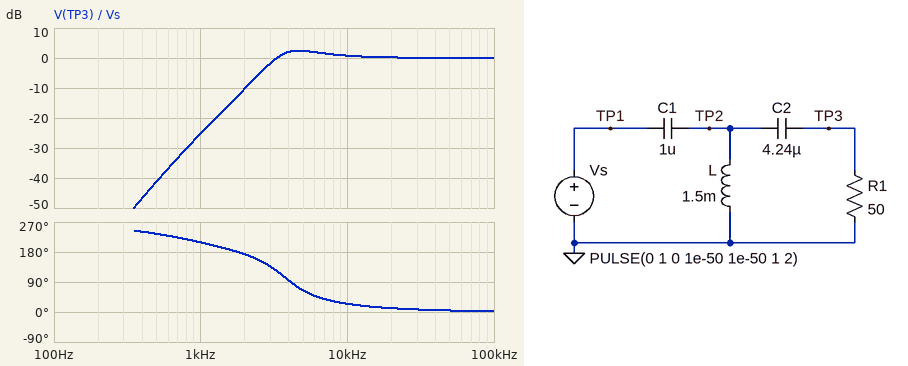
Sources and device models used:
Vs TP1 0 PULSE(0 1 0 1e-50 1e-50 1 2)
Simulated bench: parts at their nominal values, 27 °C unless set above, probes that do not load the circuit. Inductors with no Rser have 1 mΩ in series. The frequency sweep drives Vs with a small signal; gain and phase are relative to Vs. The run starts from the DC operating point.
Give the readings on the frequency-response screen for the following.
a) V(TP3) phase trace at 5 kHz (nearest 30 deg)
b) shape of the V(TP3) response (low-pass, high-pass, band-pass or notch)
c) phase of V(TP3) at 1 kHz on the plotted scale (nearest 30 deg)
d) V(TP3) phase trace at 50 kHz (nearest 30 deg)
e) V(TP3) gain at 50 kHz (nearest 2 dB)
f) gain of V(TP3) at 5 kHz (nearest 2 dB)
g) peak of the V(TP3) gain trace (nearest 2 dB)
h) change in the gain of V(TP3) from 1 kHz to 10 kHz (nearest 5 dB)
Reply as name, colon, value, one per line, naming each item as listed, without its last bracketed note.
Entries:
V(TP3) phase trace at 5 kHz: 60 deg
shape of the V(TP3) response: high-pass
phase of V(TP3) at 1 kHz on the plotted scale: 210 deg
V(TP3) phase trace at 50 kHz: 0 deg
V(TP3) gain at 50 kHz: 0 dB
gain of V(TP3) at 5 kHz: 2 dB
peak of the V(TP3) gain trace: 2 dB
change in the gain of V(TP3) from 1 kHz to 10 kHz: 25 dB
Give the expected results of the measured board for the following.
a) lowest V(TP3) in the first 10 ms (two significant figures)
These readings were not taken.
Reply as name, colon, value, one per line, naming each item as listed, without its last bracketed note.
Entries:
lowest V(TP3) in the first 10 ms: -390 mV
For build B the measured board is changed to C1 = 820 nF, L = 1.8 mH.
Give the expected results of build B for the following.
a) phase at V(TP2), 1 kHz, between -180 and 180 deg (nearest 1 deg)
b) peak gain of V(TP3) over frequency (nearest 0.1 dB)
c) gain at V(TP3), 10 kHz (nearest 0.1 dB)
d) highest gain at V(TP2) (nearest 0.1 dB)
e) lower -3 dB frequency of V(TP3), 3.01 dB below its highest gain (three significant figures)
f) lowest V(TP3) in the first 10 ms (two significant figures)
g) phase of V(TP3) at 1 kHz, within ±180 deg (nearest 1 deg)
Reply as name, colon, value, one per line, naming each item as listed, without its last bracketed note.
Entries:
phase at V(TP2), 1 kHz, between -180 and 180 deg: 170 deg
peak gain of V(TP3) over frequency: 1.1 dB
gain at V(TP3), 10 kHz: 0.5 dB
highest gain at V(TP2): 1.2 dB
lower -3 dB frequency of V(TP3), 3.01 dB below its highest gain: 3.22 kHz
lowest V(TP3) in the first 10 ms: -340 mV
phase of V(TP3) at 1 kHz, within ±180 deg: -153 deg
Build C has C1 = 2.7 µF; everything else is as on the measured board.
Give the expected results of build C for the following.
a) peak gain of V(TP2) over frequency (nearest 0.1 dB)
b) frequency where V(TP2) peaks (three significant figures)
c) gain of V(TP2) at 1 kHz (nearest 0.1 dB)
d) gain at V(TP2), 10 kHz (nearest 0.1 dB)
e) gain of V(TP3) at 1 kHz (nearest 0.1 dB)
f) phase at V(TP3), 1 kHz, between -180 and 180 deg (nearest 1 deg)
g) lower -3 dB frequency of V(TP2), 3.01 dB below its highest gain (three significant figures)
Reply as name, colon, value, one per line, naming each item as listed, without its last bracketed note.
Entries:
peak gain of V(TP2) over frequency: 6.9 dB
frequency where V(TP2) peaks: 2.44 kHz
gain of V(TP2) at 1 kHz: -13.5 dB
gain at V(TP2), 10 kHz: 0.4 dB
gain of V(TP3) at 1 kHz: -15.5 dB
phase at V(TP3), 1 kHz, between -180 and 180 deg: -152 deg
lower -3 dB frequency of V(TP2), 3.01 dB below its highest gain: 2.00 kHz
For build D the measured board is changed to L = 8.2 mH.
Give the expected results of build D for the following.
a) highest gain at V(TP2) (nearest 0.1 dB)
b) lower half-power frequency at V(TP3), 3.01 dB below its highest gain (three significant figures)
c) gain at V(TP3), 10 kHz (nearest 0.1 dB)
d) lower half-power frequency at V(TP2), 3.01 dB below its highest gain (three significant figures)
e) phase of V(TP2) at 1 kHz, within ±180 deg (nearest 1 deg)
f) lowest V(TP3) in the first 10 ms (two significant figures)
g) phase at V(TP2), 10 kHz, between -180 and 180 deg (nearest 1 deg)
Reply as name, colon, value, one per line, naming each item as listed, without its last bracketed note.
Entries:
highest gain at V(TP2): 0 dB
lower half-power frequency at V(TP3), 3.01 dB below its highest gain: 2.89 kHz
gain at V(TP3), 10 kHz: -0.4 dB
lower half-power frequency at V(TP2), 3.01 dB below its highest gain: 2.65 kHz
phase of V(TP2) at 1 kHz, within ±180 deg: 105 deg
lowest V(TP3) in the first 10 ms: -180 mV
phase at V(TP2), 10 kHz, between -180 and 180 deg: 18 deg
